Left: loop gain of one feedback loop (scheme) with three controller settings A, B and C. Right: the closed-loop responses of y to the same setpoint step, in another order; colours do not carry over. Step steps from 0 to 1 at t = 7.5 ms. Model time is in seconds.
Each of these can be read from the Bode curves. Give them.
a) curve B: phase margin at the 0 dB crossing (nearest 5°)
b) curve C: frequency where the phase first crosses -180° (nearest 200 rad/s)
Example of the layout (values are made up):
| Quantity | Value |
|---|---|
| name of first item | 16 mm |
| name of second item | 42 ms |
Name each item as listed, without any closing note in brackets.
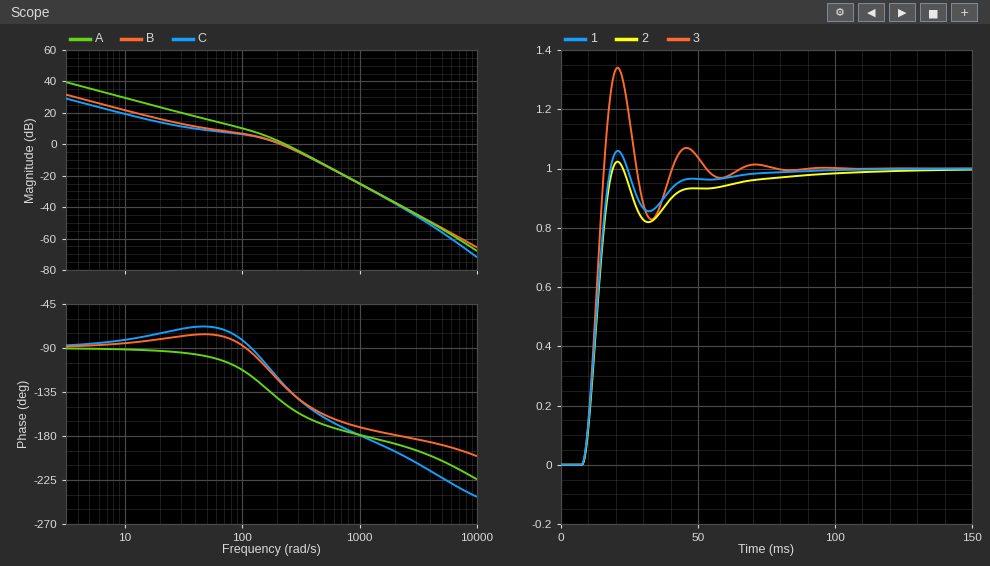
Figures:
| Quantity | Value |
|---|---|
| curve B: phase margin at the 0 dB crossing | 55° |
| curve C: frequency where the phase first crosses -180° | 1000 rad/s |
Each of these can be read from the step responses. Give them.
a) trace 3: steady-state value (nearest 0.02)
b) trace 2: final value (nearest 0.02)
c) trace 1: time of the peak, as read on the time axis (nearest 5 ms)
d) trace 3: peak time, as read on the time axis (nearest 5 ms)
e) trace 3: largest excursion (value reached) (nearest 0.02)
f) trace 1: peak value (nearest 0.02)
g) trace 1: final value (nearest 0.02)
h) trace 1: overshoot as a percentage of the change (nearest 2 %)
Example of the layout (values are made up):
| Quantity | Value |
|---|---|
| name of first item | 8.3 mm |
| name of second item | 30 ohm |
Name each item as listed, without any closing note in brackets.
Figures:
| Quantity | Value |
|---|---|
| trace 3: steady-state value | 1.00 |
| trace 2: final value | 1.00 |
| trace 1: time of the peak, as read on the time axis | 20 ms |
| trace 3: peak time, as read on the time axis | 20 ms |
| trace 3: largest excursion (value reached) | 1.34 |
| trace 1: peak value | 1.06 |
| trace 1: final value | 1.00 |
| trace 1: overshoot as a percentage of the change | 6 % |
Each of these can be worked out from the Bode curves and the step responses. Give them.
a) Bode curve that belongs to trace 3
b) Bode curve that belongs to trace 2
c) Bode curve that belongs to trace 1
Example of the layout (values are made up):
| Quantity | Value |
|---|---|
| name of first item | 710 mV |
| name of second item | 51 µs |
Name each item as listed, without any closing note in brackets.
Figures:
| Quantity | Value |
|---|---|
| Bode curve that belongs to trace 3 | A |
| Bode curve that belongs to trace 2 | C |
| Bode curve that belongs to trace 1 | B |
